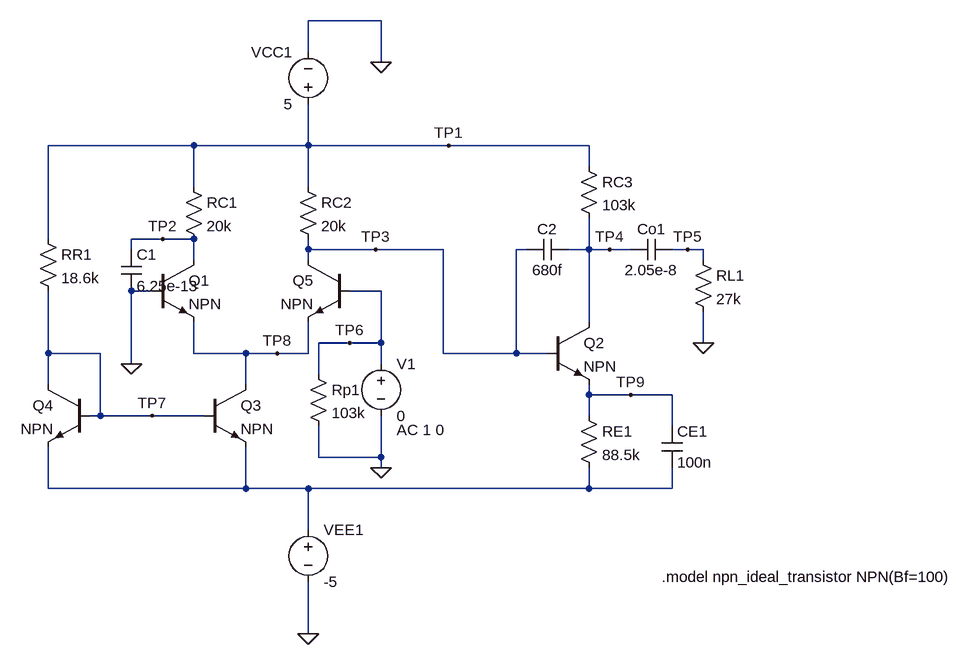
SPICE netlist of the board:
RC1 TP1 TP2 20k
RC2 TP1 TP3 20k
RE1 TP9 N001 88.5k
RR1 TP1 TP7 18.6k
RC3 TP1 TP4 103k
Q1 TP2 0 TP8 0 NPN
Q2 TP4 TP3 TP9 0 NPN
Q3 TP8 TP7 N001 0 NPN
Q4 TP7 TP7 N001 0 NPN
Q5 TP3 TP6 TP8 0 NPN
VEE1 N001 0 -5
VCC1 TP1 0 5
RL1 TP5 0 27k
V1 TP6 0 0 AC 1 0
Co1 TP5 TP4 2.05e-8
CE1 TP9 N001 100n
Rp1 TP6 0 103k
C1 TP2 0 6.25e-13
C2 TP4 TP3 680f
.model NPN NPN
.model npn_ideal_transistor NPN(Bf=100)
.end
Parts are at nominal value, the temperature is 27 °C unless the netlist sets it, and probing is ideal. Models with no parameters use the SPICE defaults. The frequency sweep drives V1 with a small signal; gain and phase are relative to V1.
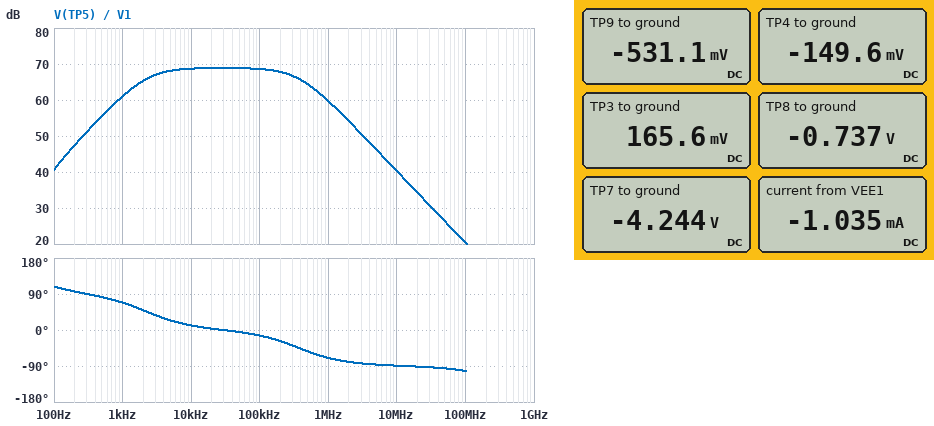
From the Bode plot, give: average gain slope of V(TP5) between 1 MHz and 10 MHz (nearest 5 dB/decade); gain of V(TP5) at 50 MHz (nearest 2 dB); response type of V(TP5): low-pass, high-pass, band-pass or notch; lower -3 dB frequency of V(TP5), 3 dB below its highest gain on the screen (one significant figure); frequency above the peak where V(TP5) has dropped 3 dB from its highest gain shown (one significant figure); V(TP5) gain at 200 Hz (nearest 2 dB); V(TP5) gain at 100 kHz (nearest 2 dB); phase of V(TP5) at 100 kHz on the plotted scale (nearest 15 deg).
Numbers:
-20 dB/decade
26 dB
band-pass
2 kHz
400 kHz
48 dB
68 dB
-15 deg
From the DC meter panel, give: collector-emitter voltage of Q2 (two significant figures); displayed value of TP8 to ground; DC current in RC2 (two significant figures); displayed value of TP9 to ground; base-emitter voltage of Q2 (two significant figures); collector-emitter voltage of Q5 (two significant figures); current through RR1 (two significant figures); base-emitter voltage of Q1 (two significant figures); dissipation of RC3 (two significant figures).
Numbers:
380 mV
-0.737 V
240 µA
-531.1 mV
700 mV
900 mV
500 µA
740 mV
260 µW
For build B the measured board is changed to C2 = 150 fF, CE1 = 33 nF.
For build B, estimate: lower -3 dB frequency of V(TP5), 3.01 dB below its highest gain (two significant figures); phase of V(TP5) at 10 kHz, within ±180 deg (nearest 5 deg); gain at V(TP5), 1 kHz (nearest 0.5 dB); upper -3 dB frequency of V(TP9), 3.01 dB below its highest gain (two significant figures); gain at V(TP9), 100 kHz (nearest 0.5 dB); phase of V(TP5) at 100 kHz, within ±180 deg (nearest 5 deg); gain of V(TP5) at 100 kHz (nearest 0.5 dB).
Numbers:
6.8 kHz
35 deg
52.0 dB
6.9 kHz
16.0 dB
0 deg
69.0 dB
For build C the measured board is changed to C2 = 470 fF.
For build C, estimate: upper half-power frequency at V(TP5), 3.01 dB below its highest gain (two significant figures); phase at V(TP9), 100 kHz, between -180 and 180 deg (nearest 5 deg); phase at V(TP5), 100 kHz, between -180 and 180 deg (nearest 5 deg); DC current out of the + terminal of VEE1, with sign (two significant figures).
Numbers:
540 kHz
80 deg
-10 deg
-1.0 mA
